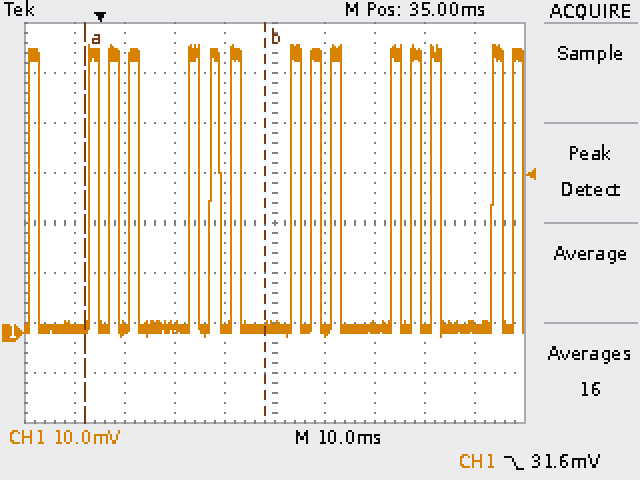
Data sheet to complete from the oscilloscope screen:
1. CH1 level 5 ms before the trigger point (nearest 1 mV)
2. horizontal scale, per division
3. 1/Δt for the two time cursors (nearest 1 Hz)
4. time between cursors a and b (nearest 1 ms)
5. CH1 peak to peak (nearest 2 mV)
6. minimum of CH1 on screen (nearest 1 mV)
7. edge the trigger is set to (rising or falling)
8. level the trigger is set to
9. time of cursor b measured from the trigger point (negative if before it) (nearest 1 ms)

1 mV
10 ms
28 Hz
36 ms
58 mV
-1 mV
falling
31.6 mV
+33 ms
